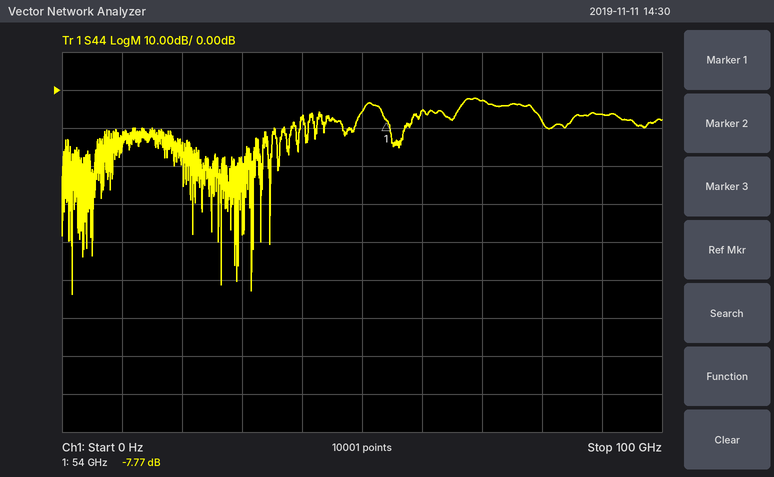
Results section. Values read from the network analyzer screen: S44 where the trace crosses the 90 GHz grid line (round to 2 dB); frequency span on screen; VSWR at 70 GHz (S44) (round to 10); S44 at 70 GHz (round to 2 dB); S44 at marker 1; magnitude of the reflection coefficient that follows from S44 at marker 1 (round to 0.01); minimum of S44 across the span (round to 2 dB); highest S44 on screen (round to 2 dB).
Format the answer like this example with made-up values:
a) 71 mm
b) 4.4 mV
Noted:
a) -6 dB
b) 100 GHz
c) 10
d) -2 dB
e) -7.77 dB
f) 0.41
g) -54 dB
h) -2 dB
